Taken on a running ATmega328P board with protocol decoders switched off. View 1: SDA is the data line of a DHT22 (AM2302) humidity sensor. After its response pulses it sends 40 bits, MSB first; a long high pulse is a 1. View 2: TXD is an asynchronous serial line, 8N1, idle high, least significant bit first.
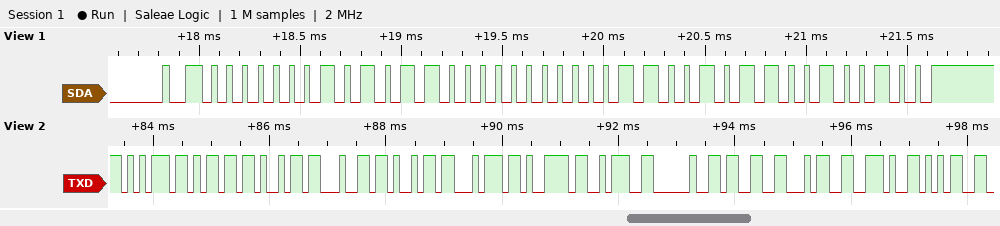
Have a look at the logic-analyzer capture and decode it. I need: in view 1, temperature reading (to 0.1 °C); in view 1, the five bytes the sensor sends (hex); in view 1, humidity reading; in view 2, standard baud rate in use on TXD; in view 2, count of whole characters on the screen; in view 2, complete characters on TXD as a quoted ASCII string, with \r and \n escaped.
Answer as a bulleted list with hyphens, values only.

- 20.3 °C
- 01 58 00 CB 24
- 34.4 %
- 9600 baud
- 13
- "umidity: 34.5"
